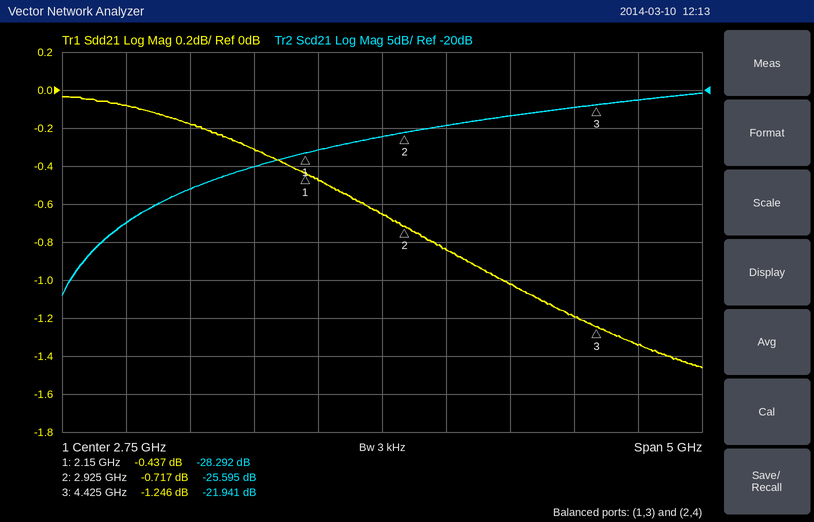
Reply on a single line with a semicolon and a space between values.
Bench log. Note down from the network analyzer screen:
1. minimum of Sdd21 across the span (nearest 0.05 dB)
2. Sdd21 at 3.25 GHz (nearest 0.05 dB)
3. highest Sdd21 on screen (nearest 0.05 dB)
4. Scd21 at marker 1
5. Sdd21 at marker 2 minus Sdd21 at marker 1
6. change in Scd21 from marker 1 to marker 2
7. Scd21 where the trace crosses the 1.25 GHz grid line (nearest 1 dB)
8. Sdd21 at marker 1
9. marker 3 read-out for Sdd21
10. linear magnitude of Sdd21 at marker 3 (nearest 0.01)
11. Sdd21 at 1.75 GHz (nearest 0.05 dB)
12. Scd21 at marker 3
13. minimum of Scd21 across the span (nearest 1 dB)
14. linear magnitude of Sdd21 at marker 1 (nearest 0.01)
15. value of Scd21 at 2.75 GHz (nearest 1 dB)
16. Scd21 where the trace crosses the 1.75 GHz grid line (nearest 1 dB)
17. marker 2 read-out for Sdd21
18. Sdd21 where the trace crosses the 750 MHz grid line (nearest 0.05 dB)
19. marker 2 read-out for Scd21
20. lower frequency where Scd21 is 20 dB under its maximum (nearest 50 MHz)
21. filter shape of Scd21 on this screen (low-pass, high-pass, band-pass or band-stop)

-1.45 dB; -0.85 dB; -0.05 dB; -28.292 dB; -0.280 dB; 2.697 dB; -33 dB; -0.437 dB; -1.246 dB; 0.87; -0.30 dB; -21.941 dB; -47 dB; 0.95; -26 dB; -30 dB; -0.717 dB; -0.10 dB; -25.595 dB; 550 MHz; high-pass
